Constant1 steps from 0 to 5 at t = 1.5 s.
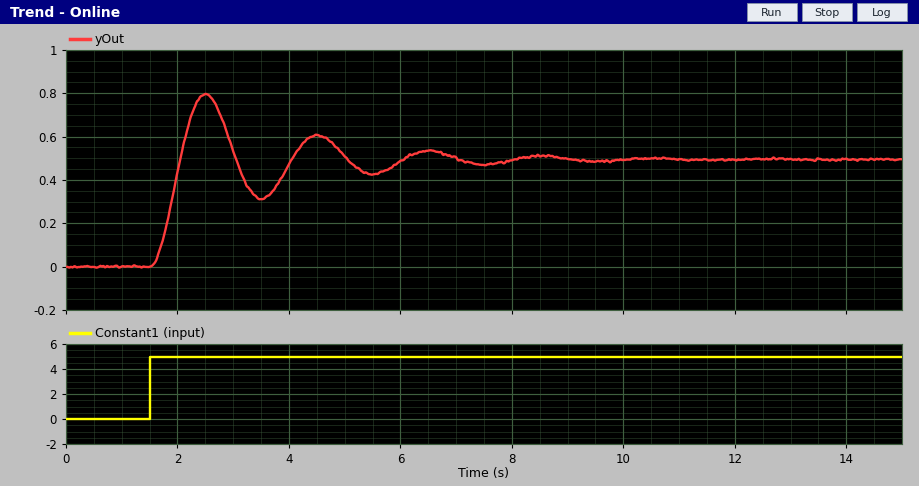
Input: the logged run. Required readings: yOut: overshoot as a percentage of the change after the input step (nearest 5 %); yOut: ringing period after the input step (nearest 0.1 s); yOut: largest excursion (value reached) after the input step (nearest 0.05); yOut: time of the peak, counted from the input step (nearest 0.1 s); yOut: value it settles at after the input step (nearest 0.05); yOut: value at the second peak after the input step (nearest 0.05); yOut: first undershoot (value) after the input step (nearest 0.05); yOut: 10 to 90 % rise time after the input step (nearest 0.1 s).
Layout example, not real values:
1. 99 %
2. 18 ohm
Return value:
1. 60 %
2. 2.0 s
3. 0.80
4. 1.0 s
5. 0.50
6. 0.60
7. 0.30
8. 0.4 s
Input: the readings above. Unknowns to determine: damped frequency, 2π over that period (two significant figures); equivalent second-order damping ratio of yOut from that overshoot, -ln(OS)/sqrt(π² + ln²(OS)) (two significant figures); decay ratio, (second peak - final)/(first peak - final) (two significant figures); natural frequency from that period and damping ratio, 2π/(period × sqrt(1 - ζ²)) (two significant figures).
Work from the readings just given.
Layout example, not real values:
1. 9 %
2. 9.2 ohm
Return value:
1. 3.1 rad/s
2. 0.16
3. 0.33
4. 3.2 rad/s
